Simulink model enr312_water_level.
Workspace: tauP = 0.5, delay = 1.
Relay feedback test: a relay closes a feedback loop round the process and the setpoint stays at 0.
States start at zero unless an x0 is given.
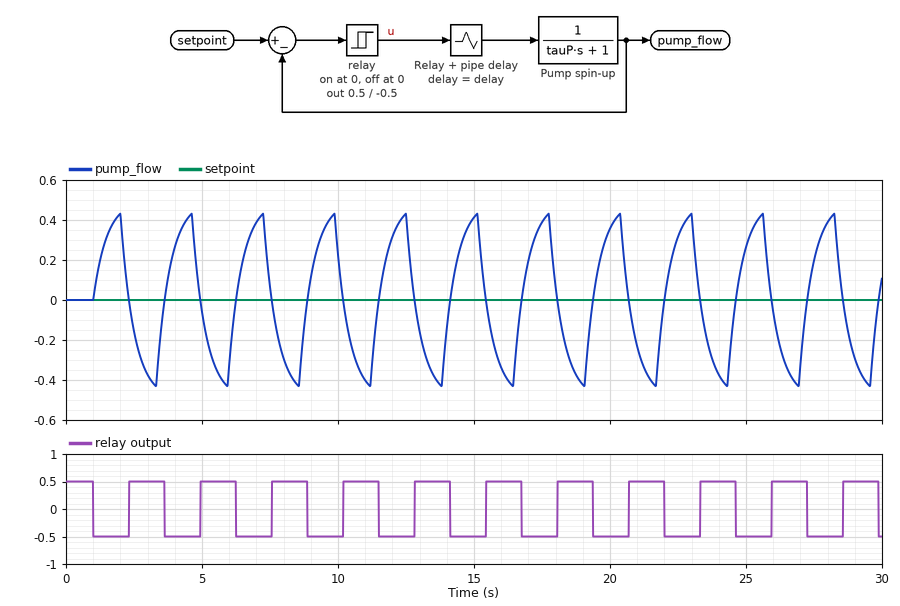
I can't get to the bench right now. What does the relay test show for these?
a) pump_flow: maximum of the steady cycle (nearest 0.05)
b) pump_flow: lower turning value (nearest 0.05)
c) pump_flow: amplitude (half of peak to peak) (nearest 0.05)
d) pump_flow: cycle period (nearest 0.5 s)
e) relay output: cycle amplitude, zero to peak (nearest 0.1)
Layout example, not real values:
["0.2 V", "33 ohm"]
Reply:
["0.45", "-0.45", "0.45", "2.5 s", "0.5"]
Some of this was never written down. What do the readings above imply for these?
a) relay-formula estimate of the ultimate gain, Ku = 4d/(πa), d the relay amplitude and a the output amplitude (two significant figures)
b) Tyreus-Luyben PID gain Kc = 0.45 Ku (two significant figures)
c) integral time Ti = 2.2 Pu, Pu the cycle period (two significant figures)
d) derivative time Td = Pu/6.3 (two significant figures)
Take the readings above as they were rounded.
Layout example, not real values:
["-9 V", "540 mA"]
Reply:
["1.4", "0.63", "5.5 s", "0.40 s"]
